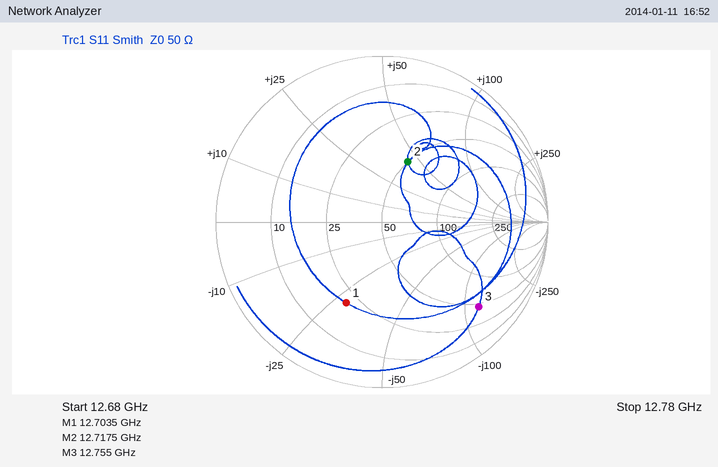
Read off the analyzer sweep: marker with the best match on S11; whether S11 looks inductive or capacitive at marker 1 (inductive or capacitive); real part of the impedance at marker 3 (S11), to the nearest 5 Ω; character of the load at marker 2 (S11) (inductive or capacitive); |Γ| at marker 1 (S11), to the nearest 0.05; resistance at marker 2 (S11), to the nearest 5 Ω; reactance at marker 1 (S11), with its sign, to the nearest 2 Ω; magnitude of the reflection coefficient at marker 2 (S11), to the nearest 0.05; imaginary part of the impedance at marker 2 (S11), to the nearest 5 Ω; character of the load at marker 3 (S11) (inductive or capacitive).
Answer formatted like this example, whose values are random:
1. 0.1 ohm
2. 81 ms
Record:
1. marker 2
2. capacitive
3. 45 Ω
4. inductive
5. 0.55
6. 50 Ω
7. -28 Ω
8. 0.40
9. +45 Ω
10. capacitive
